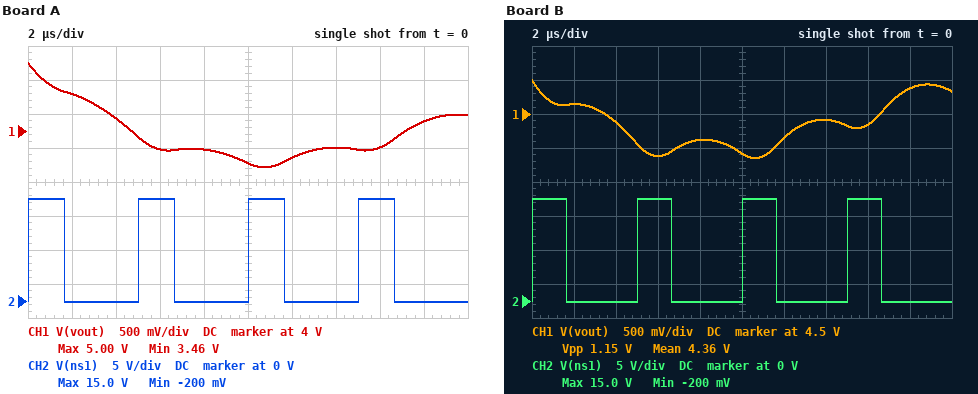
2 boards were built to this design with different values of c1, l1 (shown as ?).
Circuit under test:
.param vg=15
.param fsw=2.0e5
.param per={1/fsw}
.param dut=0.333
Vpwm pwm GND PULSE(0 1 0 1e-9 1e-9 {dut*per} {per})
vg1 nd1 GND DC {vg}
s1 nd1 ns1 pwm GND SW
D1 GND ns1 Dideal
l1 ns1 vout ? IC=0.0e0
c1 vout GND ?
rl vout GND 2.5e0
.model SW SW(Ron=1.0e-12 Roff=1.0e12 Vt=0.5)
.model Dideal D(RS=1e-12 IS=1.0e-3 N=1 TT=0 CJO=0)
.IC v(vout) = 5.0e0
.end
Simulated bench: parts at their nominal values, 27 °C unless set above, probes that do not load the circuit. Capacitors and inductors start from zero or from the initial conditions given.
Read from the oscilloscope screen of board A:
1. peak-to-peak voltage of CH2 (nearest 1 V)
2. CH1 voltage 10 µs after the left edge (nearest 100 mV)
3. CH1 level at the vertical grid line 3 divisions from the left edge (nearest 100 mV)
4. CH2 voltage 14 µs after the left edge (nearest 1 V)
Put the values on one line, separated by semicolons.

15 V; 3.5 V; 3.7 V; 0 V
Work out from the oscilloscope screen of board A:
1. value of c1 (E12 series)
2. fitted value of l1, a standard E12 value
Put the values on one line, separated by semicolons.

4.7 µF; 12 µH
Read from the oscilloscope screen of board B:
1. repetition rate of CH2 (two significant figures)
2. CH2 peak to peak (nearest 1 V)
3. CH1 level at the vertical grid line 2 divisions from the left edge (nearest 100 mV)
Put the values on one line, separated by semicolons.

200 kHz; 15 V; 4.4 V
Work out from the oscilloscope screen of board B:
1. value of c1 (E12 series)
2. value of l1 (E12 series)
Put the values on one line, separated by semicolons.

3.9 µF; 8.2 µH
